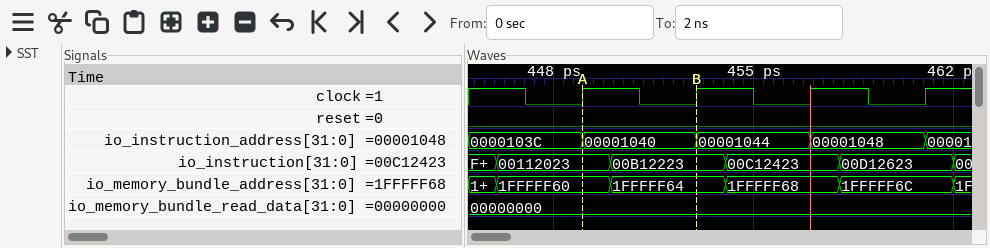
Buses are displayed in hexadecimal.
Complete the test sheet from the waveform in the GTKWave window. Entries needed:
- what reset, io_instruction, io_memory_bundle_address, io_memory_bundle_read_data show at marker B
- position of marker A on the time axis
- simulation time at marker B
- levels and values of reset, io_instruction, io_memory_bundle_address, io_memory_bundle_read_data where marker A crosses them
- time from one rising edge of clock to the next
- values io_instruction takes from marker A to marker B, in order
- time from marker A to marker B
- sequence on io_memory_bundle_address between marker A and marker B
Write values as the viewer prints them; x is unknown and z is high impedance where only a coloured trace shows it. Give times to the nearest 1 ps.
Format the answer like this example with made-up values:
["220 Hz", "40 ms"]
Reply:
["reset=0, io_instruction=00B12223, io_memory_bundle_address=1FFFFF64, io_memory_bundle_read_data=00000000", "449 ps", "453 ps", "reset=0, io_instruction=00112023, io_memory_bundle_address=1FFFFF60, io_memory_bundle_read_data=00000000", "4 ps", "00112023, 00B12223", "4 ps", "1FFFFF60, 1FFFFF64"]
